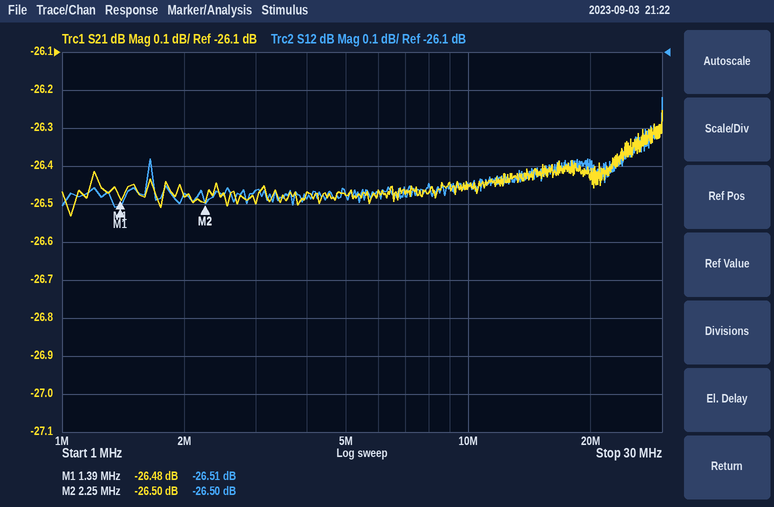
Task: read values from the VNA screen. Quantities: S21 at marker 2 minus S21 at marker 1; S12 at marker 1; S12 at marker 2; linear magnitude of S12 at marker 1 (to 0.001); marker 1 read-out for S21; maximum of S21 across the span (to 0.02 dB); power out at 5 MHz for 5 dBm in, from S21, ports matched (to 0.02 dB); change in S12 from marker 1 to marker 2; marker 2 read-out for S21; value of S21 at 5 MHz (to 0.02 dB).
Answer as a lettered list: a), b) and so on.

a) -0.02 dB
b) -26.51 dB
c) -26.50 dB
d) 0.047
e) -26.48 dB
f) -26.26 dB
g) -21.48 dBm
h) 0.01 dB
i) -26.50 dB
j) -26.48 dB
